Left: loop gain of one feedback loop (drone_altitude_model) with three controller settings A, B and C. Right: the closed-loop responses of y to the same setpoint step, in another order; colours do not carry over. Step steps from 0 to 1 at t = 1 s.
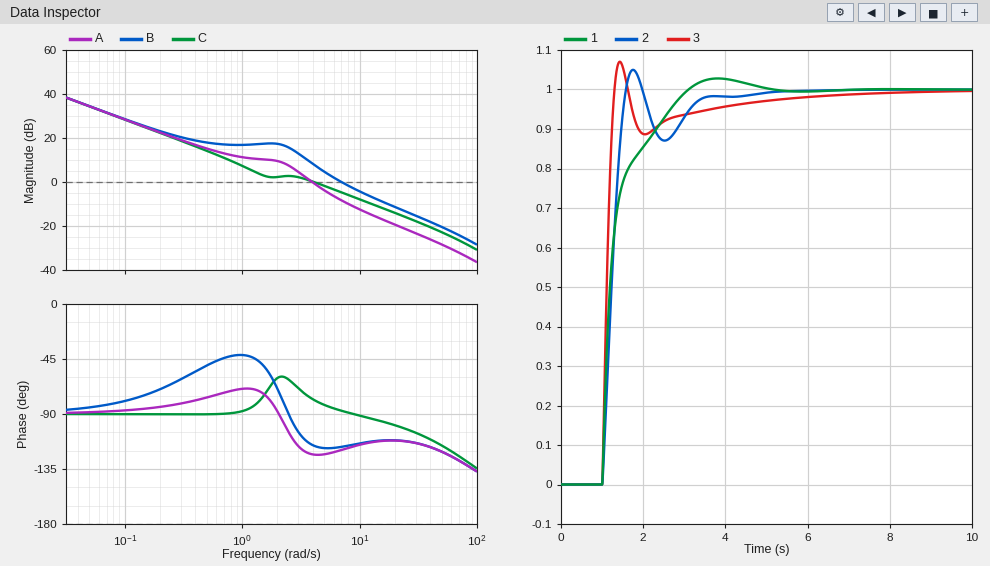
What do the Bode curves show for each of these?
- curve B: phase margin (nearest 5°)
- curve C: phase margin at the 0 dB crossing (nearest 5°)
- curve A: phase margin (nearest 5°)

65°
100°
55°
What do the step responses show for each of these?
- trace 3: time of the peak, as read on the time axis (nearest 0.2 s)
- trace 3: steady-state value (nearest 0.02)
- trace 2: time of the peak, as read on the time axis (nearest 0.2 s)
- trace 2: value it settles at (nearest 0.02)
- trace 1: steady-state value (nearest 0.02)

1.4 s
1.00
1.8 s
1.00
1.00
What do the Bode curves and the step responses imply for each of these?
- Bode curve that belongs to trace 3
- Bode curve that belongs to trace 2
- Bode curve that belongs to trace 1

B
A
C
